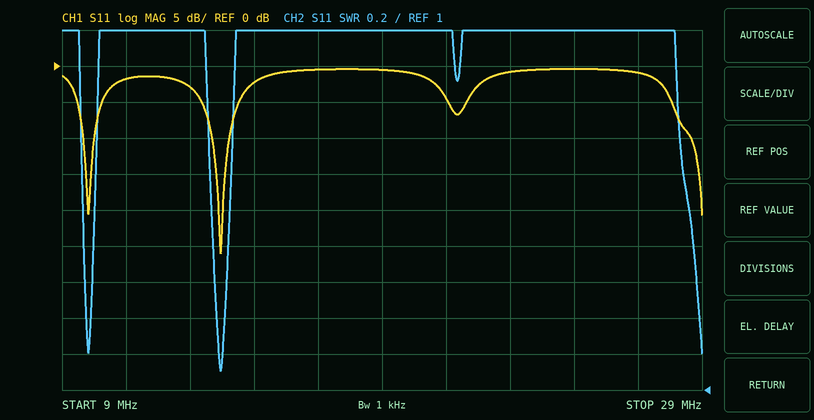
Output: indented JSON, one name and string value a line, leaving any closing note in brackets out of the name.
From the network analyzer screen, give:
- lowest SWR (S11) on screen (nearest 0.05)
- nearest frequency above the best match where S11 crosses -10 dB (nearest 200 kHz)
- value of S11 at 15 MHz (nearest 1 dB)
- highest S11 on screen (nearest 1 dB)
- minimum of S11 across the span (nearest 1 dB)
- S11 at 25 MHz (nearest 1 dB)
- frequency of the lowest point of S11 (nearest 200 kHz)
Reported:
{
  "lowest SWR (S11) on screen": "1.10",
  "nearest frequency above the best match where S11 crosses -10 dB": "14.2 MHz",
  "value of S11 at 15 MHz": "-2 dB",
  "highest S11 on screen": "0 dB",
  "minimum of S11 across the span": "-26 dB",
  "S11 at 25 MHz": "0 dB",
  "frequency of the lowest point of S11": "14.0 MHz"
}
